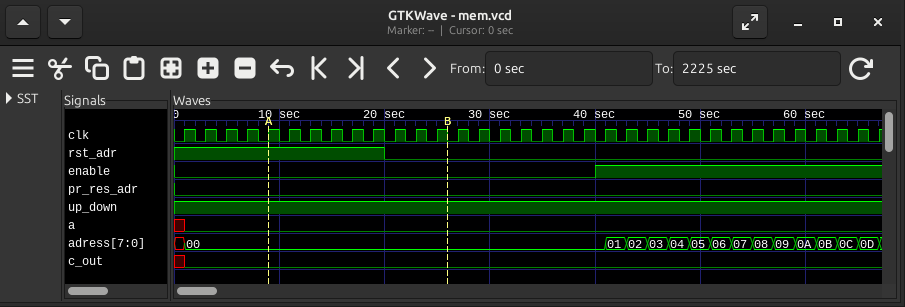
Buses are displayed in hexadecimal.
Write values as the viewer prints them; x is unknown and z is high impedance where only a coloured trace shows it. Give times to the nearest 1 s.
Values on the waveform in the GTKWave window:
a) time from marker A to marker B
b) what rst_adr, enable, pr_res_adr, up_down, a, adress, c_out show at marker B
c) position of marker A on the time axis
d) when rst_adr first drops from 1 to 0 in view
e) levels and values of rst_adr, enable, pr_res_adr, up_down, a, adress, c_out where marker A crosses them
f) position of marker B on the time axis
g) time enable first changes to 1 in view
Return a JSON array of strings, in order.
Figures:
["17 s", "rst_adr=0, enable=0, pr_res_adr=0, up_down=1, a=0, adress=00, c_out=0", "9 s", "20 s", "rst_adr=1, enable=0, pr_res_adr=0, up_down=1, a=0, adress=00, c_out=0", "26 s", "40 s"]
